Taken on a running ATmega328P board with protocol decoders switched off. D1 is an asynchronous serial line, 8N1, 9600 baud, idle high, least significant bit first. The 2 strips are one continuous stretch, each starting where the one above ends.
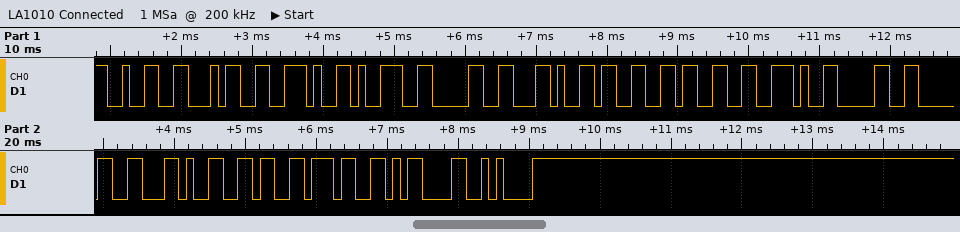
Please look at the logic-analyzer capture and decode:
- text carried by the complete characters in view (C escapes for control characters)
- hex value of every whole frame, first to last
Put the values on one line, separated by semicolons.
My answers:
"24.90,33.00,67\r\n"; 0x32 0x34 0x2E 0x39 0x30 0x2C 0x33 0x33 0x2E 0x30 0x30 0x2C 0x36 0x37 0x0D 0x0A
